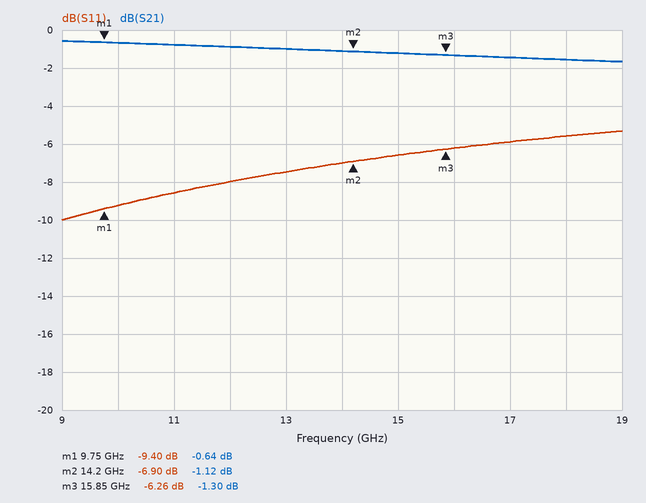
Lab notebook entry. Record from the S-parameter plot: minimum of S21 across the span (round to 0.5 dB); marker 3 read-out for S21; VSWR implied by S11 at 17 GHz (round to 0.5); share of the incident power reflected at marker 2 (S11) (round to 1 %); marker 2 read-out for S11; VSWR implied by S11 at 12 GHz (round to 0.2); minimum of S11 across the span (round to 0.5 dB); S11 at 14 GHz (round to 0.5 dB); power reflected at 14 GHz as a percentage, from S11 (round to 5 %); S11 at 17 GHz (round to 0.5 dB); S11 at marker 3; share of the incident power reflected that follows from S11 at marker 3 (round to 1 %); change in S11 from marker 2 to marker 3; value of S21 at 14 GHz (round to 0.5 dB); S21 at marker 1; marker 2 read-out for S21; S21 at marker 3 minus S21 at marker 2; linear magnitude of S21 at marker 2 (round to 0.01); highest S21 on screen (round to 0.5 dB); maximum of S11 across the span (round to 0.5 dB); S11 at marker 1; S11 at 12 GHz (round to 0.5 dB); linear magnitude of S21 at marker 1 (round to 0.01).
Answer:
-1.5 dB
-1.30 dB
3.0
20 %
-6.90 dB
2.4
-10.0 dB
-7.0 dB
20 %
-6.0 dB
-6.26 dB
24 %
0.64 dB
-1.0 dB
-0.64 dB
-1.12 dB
-0.18 dB
0.88
-0.5 dB
-5.5 dB
-9.40 dB
-8.0 dB
0.93
